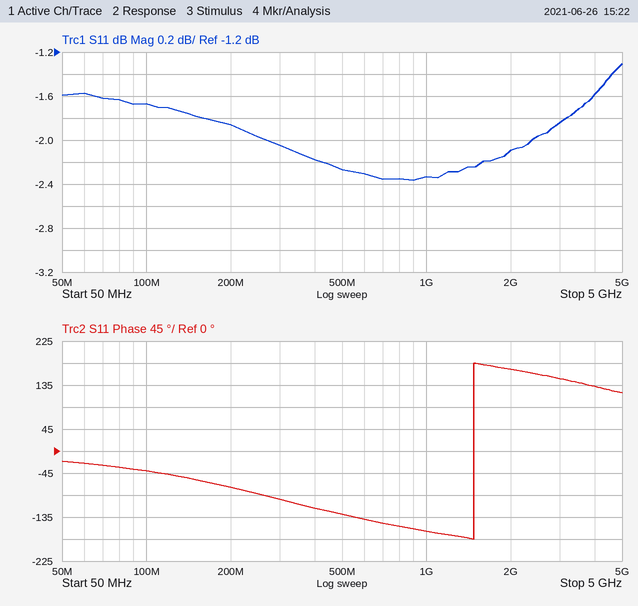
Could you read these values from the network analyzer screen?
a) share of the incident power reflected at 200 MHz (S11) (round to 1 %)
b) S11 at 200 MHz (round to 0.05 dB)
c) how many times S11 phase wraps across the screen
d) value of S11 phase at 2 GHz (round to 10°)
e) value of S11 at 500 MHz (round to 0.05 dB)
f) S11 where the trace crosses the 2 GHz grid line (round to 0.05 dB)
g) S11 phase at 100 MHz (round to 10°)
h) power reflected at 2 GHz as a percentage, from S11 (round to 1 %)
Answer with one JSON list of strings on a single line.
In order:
["65 %", "-1.85 dB", "1", "170°", "-2.25 dB", "-2.10 dB", "-40°", "62 %"]
